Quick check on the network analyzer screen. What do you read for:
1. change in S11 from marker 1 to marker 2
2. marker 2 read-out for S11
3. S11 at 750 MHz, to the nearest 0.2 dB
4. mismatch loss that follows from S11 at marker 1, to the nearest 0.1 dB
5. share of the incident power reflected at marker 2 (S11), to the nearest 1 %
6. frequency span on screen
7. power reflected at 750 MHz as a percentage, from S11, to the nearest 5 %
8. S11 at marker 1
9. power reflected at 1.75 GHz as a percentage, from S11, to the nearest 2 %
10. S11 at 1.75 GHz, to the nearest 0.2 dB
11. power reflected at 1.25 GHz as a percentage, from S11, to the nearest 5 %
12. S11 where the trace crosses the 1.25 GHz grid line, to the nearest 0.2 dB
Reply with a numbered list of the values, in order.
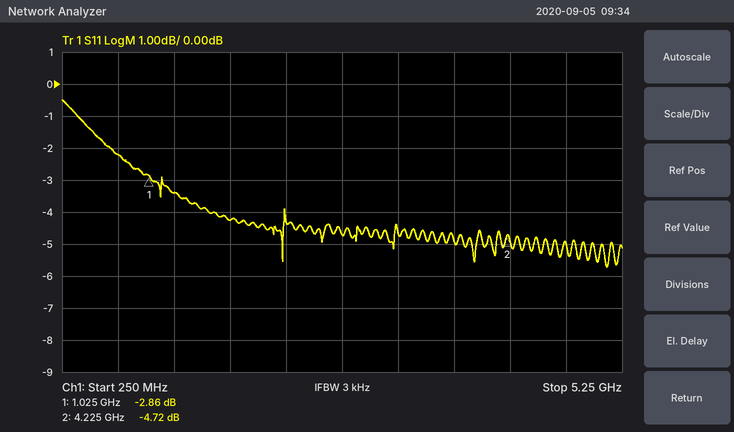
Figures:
1. -1.86 dB
2. -4.72 dB
3. -2.2 dB
4. 3.2 dB
5. 34 %
6. 5 GHz
7. 60 %
8. -2.86 dB
9. 38 %
10. -4.2 dB
11. 45 %
12. -3.4 dB
